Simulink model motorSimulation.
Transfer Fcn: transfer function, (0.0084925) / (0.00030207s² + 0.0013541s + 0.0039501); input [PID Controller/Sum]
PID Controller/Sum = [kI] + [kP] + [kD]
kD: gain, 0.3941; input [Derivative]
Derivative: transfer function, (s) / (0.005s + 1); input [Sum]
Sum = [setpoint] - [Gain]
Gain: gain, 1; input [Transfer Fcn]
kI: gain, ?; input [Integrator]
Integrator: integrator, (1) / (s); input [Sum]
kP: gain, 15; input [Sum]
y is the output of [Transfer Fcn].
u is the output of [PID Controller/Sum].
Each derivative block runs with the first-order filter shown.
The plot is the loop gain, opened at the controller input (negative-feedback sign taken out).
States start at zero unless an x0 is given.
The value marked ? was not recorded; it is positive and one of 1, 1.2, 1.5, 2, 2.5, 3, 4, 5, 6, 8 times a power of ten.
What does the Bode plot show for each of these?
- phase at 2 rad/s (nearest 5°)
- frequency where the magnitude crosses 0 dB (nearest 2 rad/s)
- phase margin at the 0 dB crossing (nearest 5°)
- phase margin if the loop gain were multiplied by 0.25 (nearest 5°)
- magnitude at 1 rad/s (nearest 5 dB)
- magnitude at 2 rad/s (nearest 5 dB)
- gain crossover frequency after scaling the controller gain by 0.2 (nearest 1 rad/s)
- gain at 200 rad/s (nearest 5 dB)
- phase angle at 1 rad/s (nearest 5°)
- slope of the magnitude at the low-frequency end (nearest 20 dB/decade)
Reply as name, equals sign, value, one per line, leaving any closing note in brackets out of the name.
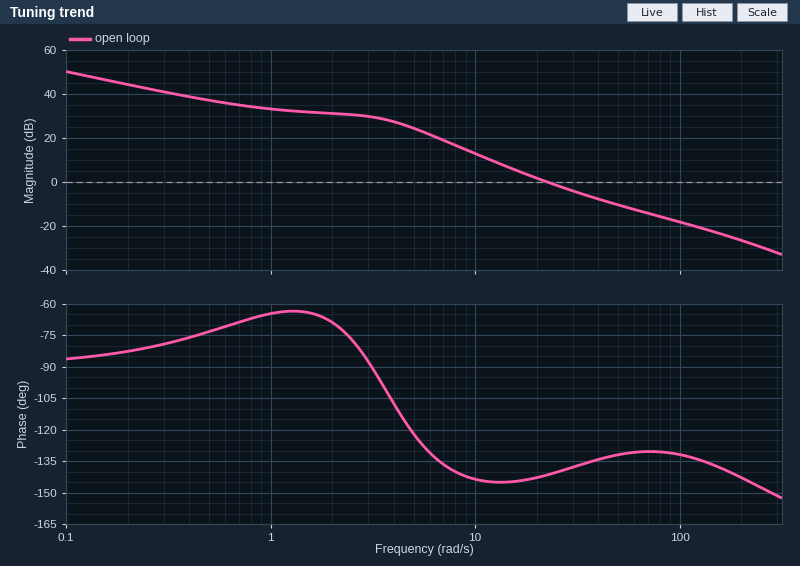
phase at 2 rad/s = -70°
frequency where the magnitude crosses 0 dB = 22 rad/s
phase margin at the 0 dB crossing = 40°
phase margin if the loop gain were multiplied by 0.25 = 35°
magnitude at 1 rad/s = 35 dB
magnitude at 2 rad/s = 30 dB
gain crossover frequency after scaling the controller gain by 0.2 = 9 rad/s
gain at 200 rad/s = -25 dB
phase angle at 1 rad/s = -65°
slope of the magnitude at the low-frequency end = -20 dB/decade
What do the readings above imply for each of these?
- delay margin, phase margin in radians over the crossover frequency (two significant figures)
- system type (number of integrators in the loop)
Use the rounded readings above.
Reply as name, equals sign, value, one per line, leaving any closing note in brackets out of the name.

delay margin, phase margin in radians over the crossover frequency = 0.032 s
system type = 1
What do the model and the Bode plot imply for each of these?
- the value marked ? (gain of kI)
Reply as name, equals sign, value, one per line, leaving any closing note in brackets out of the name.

the value marked ? = 15
